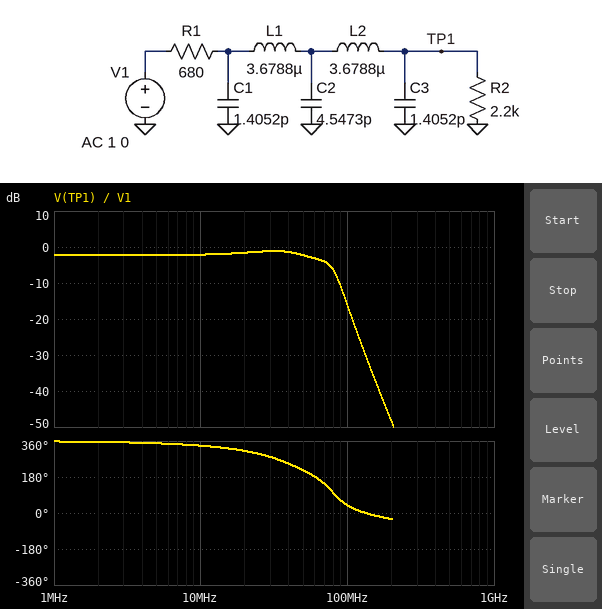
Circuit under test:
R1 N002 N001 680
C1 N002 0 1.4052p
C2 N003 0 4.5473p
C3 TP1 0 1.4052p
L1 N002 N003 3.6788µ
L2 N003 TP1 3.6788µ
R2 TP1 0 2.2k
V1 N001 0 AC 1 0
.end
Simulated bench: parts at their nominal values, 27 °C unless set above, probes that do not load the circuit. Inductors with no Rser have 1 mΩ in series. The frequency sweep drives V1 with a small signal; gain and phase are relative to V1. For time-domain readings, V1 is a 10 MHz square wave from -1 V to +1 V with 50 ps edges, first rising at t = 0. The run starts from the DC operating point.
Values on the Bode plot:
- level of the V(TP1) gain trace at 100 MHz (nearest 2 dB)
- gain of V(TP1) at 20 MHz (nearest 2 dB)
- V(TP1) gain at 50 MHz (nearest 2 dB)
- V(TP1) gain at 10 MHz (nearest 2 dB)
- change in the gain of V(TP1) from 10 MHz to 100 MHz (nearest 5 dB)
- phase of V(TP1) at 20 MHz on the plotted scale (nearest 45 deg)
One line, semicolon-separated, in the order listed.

-16 dB; -2 dB; -2 dB; -2 dB; -15 dB; 315 deg
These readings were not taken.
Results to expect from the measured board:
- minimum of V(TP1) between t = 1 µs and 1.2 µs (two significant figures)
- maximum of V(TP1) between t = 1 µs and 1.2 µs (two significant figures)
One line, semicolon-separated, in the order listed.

-1.1 V; 1.1 V
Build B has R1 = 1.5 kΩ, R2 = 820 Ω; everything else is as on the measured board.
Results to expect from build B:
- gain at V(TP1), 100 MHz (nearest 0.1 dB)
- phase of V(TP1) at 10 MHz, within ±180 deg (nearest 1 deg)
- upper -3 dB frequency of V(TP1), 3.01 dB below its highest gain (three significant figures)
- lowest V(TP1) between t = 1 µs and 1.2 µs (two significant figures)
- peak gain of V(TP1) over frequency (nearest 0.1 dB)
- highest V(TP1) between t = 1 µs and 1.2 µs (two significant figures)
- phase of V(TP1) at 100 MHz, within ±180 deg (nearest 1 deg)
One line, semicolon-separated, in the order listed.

-23.8 dB; -26 deg; 71.1 MHz; -460 mV; -8.7 dB; 460 mV; 46 deg
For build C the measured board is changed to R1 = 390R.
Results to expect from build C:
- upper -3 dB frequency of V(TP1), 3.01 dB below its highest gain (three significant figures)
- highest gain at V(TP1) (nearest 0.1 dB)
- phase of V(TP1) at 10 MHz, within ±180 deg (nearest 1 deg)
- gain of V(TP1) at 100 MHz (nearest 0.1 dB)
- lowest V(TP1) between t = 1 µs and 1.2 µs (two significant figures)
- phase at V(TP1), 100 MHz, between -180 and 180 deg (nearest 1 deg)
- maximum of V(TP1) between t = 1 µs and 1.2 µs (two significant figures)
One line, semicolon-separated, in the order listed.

54.7 MHz; 1.5 dB; -20 deg; -15.9 dB; -1.4 V; 44 deg; 1.4 V
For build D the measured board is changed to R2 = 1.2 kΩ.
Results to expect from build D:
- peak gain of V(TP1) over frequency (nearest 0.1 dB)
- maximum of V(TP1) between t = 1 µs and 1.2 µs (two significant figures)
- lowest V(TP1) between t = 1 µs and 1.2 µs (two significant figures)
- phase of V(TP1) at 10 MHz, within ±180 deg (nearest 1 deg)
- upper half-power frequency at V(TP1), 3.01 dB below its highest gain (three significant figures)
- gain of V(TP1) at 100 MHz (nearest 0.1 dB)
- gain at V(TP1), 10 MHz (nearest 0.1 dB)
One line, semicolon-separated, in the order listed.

-3.6 dB; 830 mV; -830 mV; -26 deg; 68.1 MHz; -20.0 dB; -3.8 dB
